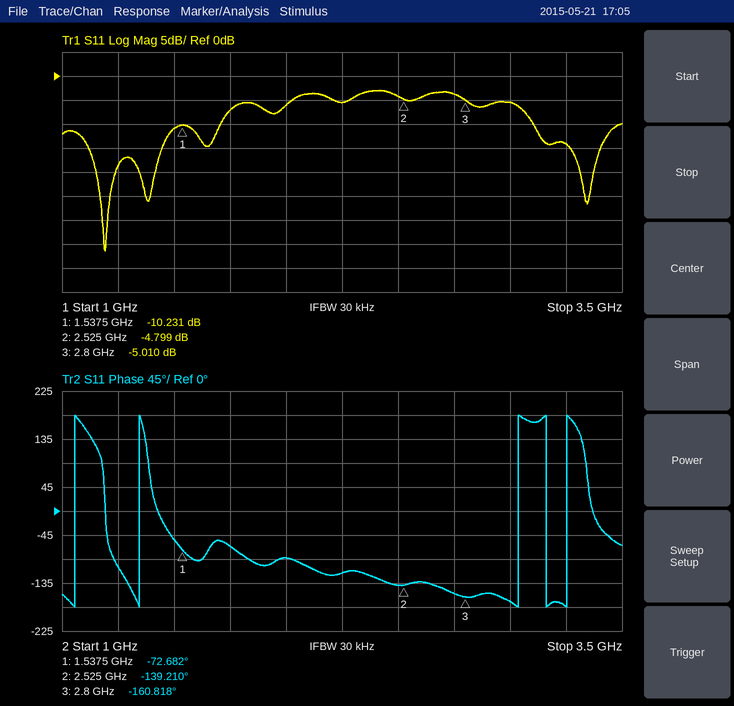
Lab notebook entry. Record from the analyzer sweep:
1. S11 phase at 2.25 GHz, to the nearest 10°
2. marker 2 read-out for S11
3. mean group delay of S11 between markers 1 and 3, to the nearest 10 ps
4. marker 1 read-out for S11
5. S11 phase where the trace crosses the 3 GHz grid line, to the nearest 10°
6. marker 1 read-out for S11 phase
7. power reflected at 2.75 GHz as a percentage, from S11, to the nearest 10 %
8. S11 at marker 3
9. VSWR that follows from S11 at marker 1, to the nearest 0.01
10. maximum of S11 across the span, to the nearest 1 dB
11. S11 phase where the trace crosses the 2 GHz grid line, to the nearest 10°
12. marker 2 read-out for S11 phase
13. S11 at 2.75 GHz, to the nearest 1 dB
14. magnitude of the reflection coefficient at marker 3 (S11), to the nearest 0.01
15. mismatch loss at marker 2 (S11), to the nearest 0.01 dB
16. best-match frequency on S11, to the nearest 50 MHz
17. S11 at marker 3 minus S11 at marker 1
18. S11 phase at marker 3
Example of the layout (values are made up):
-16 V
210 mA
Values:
-120°
-4.799 dB
190 ps
-10.231 dB
-170°
-72.682°
40 %
-5.010 dB
1.89
-3 dB
-90°
-139.210°
-4 dB
0.56
1.75 dB
1.20 GHz
5.221 dB
-160.818°
